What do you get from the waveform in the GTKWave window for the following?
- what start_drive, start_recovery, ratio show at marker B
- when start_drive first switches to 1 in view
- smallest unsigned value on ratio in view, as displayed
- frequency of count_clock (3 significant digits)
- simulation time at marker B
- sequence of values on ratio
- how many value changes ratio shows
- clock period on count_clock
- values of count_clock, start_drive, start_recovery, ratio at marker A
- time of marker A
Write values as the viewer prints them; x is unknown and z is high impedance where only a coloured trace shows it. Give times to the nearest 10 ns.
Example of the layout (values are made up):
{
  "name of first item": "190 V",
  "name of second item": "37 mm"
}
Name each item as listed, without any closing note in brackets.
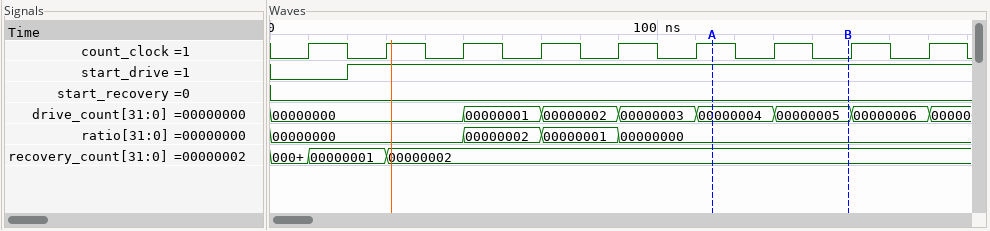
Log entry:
{
  "what start_drive, start_recovery, ratio show at marker B": "start_drive=1, start_recovery=0, ratio=00000000",
  "when start_drive first switches to 1 in view": "20 ns",
  "smallest unsigned value on ratio in view, as displayed": "00000000",
  "frequency of count_clock": "50.0 MHz",
  "simulation time at marker B": "150 ns",
  "sequence of values on ratio": "00000000, 00000002, 00000001, 00000000",
  "how many value changes ratio shows": "3",
  "clock period on count_clock": "20 ns",
  "values of count_clock, start_drive, start_recovery, ratio at marker A": "count_clock=1, start_drive=1, start_recovery=0, ratio=00000000",
  "time of marker A": "110 ns"
}
